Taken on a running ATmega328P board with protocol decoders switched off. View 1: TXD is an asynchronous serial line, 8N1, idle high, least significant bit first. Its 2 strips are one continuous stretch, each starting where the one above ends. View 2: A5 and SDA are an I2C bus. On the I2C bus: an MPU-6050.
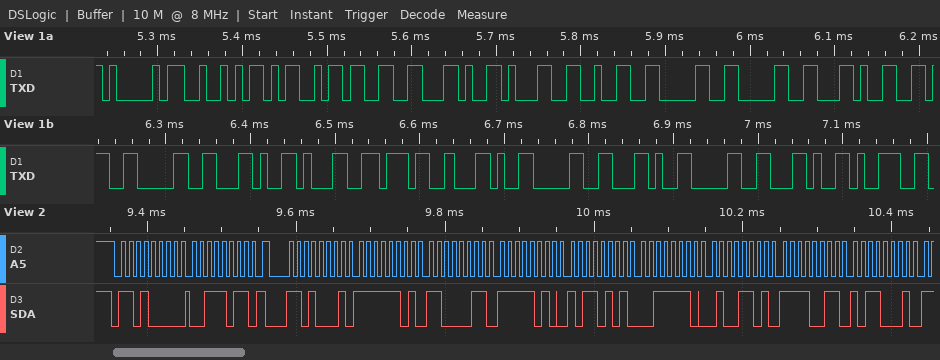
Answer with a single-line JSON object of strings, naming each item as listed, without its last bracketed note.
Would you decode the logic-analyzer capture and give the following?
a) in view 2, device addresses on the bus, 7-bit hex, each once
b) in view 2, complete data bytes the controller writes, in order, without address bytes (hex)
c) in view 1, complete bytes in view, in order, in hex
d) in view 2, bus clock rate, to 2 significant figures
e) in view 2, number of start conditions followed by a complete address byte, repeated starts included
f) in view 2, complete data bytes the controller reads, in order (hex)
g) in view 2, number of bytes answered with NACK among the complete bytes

{"in view 2, device addresses on the bus, 7-bit hex, each once": "0x68", "in view 2, complete data bytes the controller writes, in order, without address bytes": "3B", "in view 1, complete bytes in view, in order, in hex": "41 52 4D 33 2C 31 32 30 30 2C 36 30 2C 31 37 2C 30 2C 30 2C 39", "in view 2, bus clock rate, to 2 significant figures": "100 kHz", "in view 2, number of start conditions followed by a complete address byte, repeated starts included": "2", "in view 2, complete data bytes the controller reads, in order": "FD C3 FA B5 3E 4D F3 B1", "in view 2, number of bytes answered with NACK among the complete bytes": "0"}
